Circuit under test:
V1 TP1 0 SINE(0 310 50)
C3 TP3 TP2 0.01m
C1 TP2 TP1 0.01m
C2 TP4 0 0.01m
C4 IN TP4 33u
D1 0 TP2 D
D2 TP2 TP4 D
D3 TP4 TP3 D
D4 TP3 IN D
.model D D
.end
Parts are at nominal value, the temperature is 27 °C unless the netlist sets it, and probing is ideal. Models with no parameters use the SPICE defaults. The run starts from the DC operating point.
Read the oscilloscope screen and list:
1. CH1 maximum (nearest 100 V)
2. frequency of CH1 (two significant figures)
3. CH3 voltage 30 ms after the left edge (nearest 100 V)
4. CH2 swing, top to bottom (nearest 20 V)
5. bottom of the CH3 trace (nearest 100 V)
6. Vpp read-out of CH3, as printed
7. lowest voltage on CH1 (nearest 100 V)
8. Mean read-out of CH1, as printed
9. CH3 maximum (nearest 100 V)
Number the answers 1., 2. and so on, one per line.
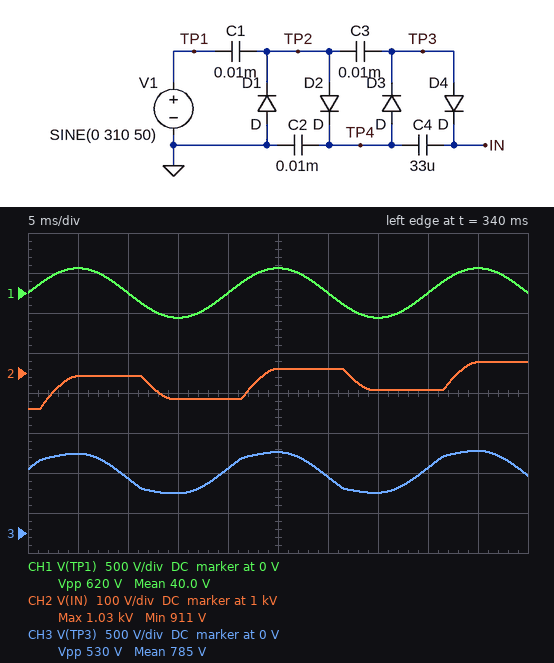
1. 300 V
2. 50 Hz
3. 700 V
4. 120 V
5. 500 V
6. 530 V
7. -300 V
8. 40.0 V
9. 1.0 kV
